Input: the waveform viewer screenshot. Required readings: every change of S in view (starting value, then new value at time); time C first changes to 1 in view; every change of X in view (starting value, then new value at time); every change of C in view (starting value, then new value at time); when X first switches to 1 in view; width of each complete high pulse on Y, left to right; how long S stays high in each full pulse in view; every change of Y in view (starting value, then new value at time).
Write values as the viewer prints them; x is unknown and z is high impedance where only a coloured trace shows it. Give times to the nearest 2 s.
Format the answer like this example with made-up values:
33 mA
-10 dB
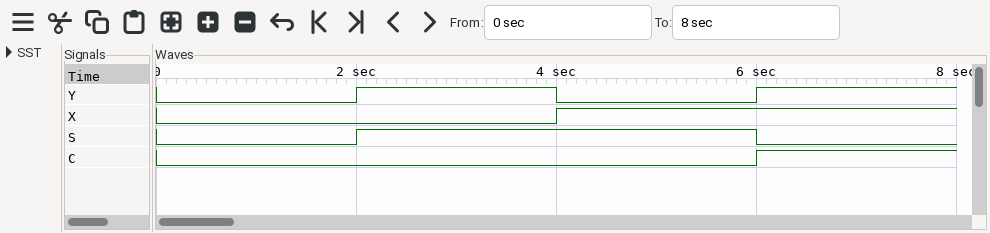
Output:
0, 1 at 2 s, 0 at 6 s
6 s
0, 1 at 4 s
0, 1 at 6 s
4 s
2 s
4 s
0, 1 at 2 s, 0 at 4 s, 1 at 6 s
